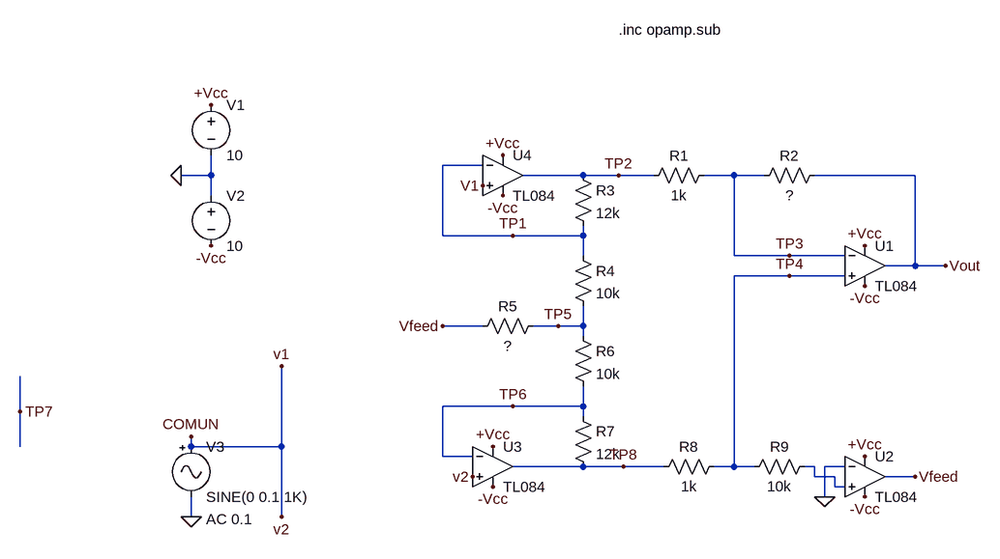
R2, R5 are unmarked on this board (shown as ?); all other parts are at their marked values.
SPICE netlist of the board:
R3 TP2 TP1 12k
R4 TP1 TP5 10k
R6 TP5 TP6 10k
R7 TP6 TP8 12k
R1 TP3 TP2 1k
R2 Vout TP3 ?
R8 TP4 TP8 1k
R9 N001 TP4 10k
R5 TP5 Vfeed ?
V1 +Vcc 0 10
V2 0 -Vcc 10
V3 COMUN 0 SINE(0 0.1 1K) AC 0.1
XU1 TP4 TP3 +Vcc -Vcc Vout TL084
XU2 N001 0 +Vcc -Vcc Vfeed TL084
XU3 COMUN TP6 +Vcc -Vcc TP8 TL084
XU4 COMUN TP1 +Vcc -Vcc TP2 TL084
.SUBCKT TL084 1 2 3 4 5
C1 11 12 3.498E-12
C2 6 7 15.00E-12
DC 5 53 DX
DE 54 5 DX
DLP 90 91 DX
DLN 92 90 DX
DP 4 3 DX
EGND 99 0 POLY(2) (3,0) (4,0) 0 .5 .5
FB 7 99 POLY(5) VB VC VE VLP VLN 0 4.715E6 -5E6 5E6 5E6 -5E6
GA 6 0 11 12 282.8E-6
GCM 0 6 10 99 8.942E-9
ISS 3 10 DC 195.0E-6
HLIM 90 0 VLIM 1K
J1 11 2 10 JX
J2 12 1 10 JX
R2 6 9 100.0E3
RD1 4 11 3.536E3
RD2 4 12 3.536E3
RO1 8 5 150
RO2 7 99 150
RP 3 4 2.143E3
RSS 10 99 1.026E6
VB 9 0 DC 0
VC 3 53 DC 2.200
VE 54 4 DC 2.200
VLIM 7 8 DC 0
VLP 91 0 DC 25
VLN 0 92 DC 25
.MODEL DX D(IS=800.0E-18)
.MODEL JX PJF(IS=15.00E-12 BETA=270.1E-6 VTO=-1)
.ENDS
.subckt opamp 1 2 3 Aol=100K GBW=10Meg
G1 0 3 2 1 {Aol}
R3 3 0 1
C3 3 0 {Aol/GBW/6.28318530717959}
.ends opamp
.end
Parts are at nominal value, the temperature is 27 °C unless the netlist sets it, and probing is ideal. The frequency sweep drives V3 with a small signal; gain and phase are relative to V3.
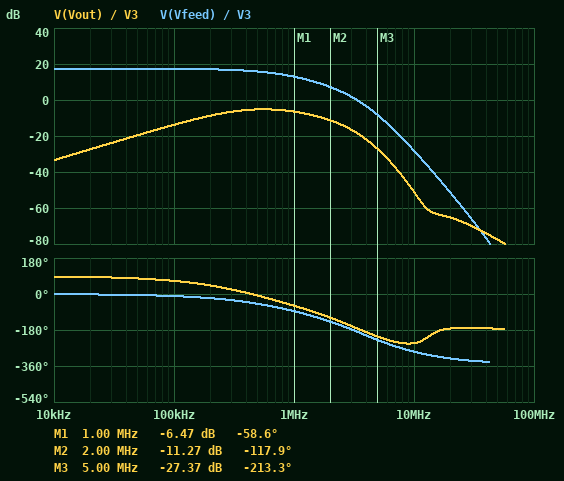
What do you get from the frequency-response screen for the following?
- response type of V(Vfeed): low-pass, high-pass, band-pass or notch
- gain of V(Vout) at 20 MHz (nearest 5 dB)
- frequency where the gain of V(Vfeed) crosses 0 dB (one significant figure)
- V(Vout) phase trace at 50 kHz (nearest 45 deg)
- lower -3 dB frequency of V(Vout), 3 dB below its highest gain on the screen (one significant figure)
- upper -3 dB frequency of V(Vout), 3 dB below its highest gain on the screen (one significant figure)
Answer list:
low-pass
-65 dB
3 MHz
90 deg
200 kHz
1 MHz
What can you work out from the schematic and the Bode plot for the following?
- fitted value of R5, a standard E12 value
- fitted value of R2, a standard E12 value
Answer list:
33 kΩ
8.2 kΩ
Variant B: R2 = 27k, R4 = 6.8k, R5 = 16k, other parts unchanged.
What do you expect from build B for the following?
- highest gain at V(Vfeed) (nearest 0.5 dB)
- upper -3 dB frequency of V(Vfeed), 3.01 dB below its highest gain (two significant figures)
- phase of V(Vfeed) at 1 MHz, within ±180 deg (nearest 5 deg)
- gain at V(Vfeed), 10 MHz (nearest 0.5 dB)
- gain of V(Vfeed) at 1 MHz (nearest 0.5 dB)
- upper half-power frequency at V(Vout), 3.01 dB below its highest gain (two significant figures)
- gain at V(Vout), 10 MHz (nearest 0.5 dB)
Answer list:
14.0 dB
1.5 MHz
-70 deg
-28.5 dB
12.5 dB
120 kHz
-58.0 dB
